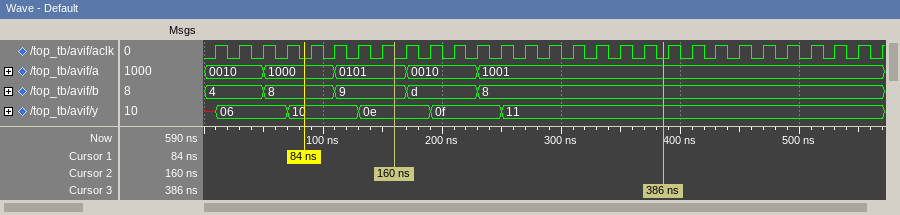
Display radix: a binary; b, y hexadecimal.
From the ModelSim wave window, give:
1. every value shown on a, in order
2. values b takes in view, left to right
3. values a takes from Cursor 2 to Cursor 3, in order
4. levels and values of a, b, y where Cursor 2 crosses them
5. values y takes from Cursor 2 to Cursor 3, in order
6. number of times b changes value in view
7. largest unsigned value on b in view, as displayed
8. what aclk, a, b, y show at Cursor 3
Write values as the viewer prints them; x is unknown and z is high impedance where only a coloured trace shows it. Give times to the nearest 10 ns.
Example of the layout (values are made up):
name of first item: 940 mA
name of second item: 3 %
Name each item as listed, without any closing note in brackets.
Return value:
every value shown on a, in order: 0010, 1000, 0101, 0010, 1001
values b takes in view, left to right: 4, 8, 9, d, 8
values a takes from Cursor 2 to Cursor 3, in order: 0101, 0010, 1001
levels and values of a, b, y where Cursor 2 crosses them: a=0101, b=9, y=0e
values y takes from Cursor 2 to Cursor 3, in order: 0e, 0f, 11
number of times b changes value in view: 4
largest unsigned value on b in view, as displayed: d
what aclk, a, b, y show at Cursor 3: aclk=0, a=1001, b=8, y=11
